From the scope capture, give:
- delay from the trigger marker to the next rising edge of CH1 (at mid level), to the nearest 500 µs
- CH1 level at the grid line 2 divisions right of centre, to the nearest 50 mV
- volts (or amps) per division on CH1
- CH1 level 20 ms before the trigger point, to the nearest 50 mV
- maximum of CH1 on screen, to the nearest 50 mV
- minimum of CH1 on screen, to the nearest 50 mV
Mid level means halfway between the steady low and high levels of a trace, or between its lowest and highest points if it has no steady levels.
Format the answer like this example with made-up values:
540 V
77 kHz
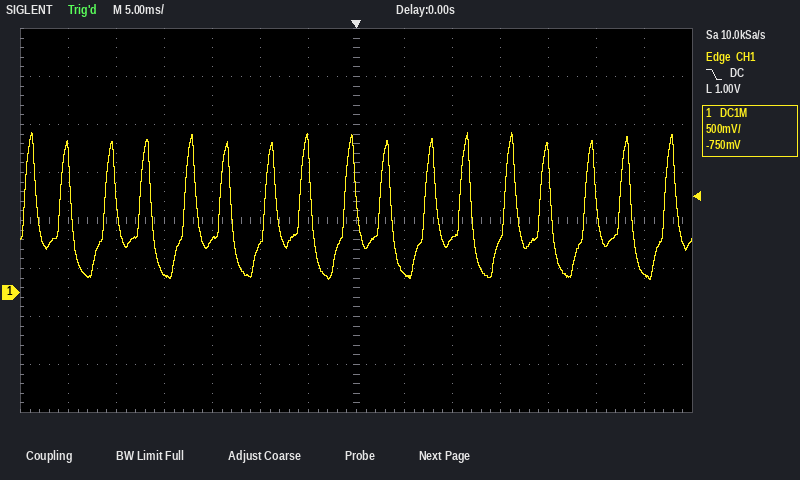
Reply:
2.5 ms
550 mV
500 mV
200 mV
1.65 V
150 mV
